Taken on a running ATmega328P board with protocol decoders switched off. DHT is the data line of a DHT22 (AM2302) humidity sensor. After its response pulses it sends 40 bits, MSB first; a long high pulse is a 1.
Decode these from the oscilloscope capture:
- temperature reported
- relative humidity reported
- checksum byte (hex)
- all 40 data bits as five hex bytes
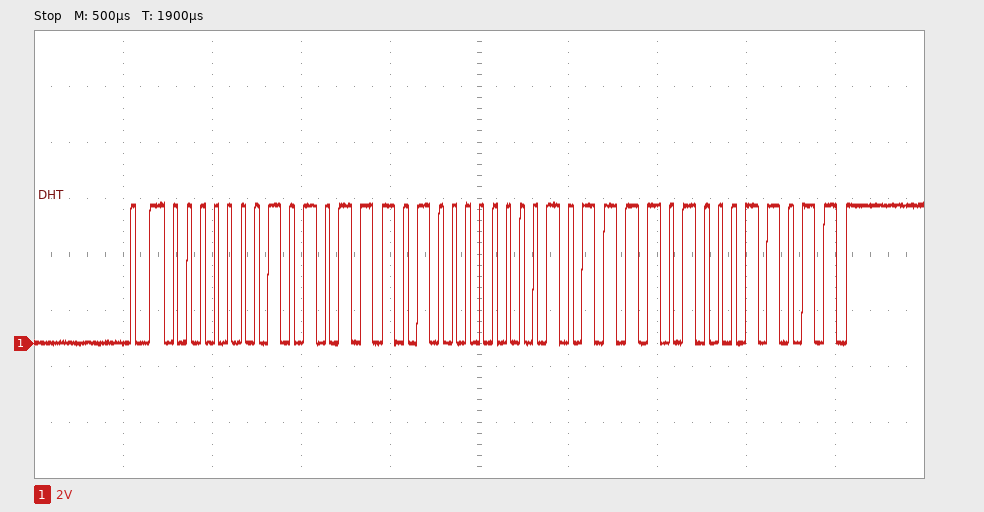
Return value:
18.9 °C
34.9 %
0x1B
01 5D 00 BD 1B
